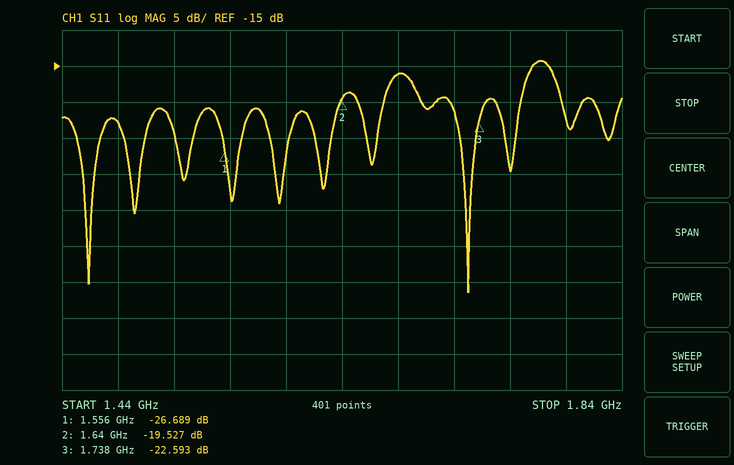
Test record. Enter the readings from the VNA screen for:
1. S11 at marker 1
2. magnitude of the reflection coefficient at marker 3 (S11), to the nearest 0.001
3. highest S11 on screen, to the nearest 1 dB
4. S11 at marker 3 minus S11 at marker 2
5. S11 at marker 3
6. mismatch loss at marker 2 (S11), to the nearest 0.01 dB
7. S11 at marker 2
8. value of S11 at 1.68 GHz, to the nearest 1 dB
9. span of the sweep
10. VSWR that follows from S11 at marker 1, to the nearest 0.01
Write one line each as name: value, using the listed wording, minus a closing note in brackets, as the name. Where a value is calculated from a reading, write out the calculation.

S11 at marker 1: -26.689 dB
magnitude of the reflection coefficient at marker 3 (S11), to the nearest 0.001: 10^(-22.593/20) ≈ 0.074
highest S11 on screen, to the nearest 1 dB: -14 dB
S11 at marker 3 minus S11 at marker 2: -22.593 − (-19.527) = -3.066 dB
S11 at marker 3: -22.593 dB
mismatch loss at marker 2 (S11), to the nearest 0.01 dB: −10 log10(1 − 10^(-19.527/10)) ≈ 0.05 dB
S11 at marker 2: -19.527 dB
value of S11 at 1.68 GHz, to the nearest 1 dB: -16 dB
span of the sweep: 400 MHz
VSWR that follows from S11 at marker 1, to the nearest 0.01: (1 + 0.0463)/(1 − 0.0463) ≈ 1.10
